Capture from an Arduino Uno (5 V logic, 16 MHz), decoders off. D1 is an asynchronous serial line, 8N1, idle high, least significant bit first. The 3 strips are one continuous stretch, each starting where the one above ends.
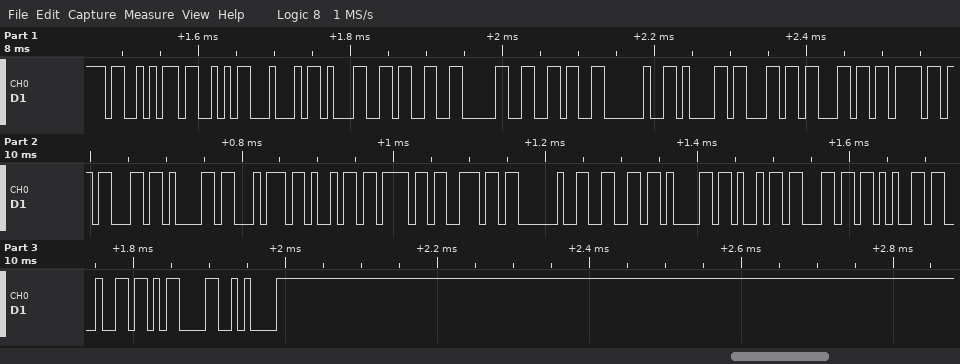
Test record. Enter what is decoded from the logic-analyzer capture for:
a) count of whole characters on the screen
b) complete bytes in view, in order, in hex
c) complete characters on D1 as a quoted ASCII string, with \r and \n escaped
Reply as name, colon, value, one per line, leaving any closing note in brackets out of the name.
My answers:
count of whole characters on the screen: 27
complete bytes in view, in order, in hex: 0x53 0x53 0x44 0x31 0x33 0x30 0x36 0x20 0x61 0x6C 0x6C 0x6F 0x63 0x61 0x74 0x69 0x6F 0x6E 0x20 0x66 0x61 0x69 0x6C 0x65 0x64 0x0D 0x0A
complete characters on D1 as a quoted ASCII string, with \r and \n escaped: "SSD1306 allocation failed\r\n"
